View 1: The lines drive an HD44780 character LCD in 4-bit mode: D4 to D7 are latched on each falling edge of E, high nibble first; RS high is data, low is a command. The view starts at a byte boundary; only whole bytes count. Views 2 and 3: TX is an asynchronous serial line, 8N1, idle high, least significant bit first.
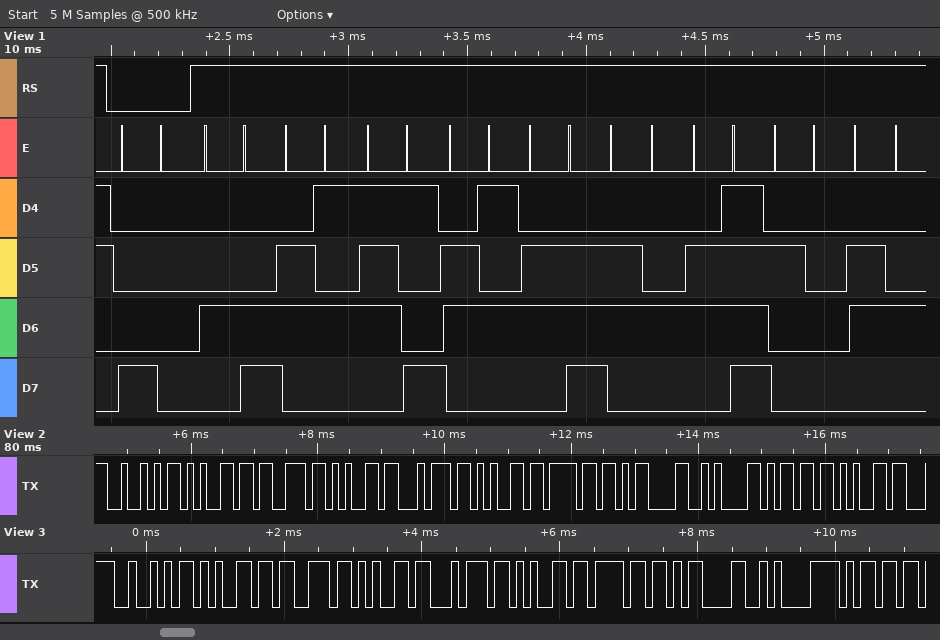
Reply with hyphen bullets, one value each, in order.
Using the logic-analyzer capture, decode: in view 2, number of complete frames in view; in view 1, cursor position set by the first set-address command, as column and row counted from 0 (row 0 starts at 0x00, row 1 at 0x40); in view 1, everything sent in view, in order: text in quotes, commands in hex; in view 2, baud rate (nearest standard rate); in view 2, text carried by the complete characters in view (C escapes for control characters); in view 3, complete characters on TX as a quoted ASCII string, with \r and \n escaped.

- 11
- column 0, row 0
- 0x80 "Leyendo d"
- 9600 baud
- "Reseteo\r\nme"
- "Reseteo\r\nm"
